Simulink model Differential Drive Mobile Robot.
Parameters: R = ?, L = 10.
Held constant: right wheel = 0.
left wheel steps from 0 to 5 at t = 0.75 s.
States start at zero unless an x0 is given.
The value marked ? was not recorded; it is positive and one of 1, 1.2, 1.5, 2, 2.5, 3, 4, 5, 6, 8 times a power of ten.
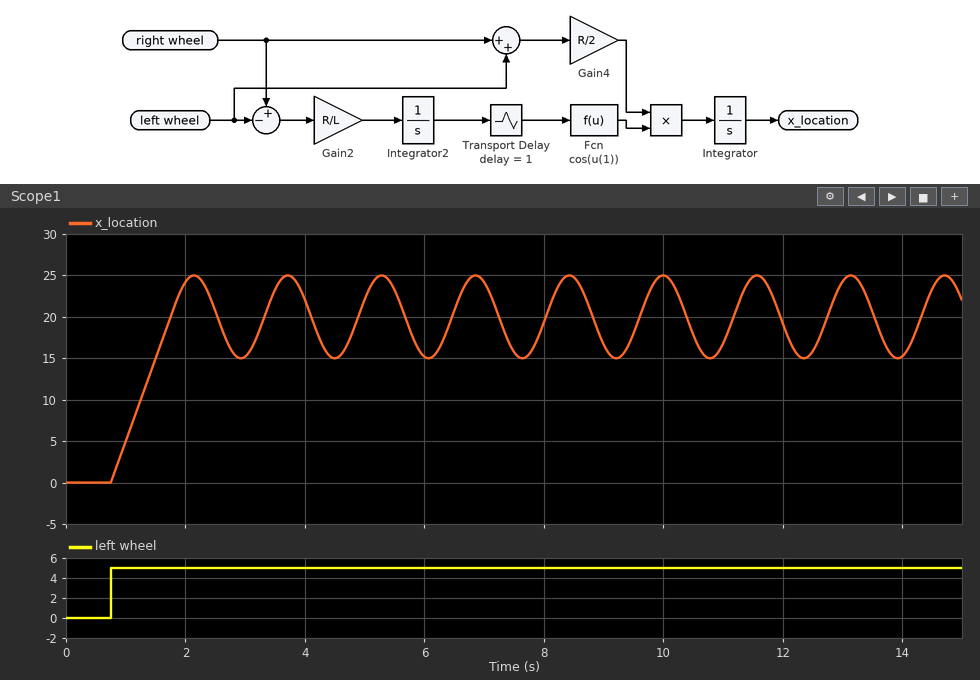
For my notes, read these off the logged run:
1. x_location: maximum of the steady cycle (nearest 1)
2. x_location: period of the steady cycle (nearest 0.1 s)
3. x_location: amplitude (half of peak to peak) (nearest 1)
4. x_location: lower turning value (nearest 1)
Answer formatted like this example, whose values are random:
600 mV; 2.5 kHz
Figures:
25; 1.6 s; 5; 15
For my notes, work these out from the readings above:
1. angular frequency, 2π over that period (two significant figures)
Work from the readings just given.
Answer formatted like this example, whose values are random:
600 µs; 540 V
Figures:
3.9 rad/s
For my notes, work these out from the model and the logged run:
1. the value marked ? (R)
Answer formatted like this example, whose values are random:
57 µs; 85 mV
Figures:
8
